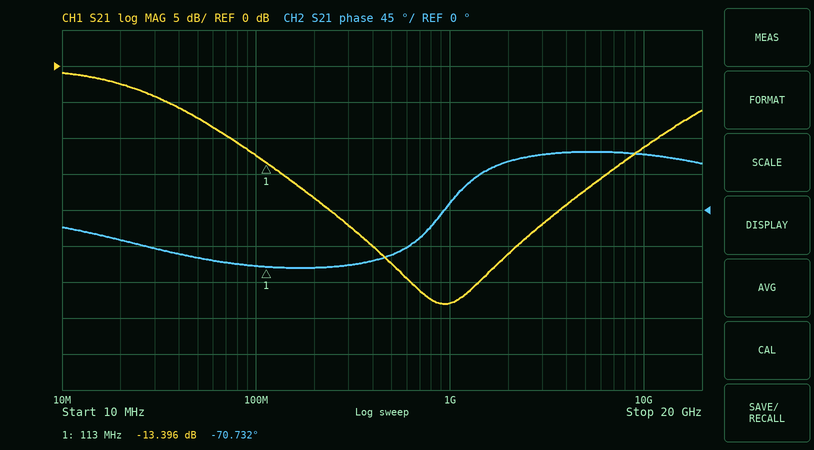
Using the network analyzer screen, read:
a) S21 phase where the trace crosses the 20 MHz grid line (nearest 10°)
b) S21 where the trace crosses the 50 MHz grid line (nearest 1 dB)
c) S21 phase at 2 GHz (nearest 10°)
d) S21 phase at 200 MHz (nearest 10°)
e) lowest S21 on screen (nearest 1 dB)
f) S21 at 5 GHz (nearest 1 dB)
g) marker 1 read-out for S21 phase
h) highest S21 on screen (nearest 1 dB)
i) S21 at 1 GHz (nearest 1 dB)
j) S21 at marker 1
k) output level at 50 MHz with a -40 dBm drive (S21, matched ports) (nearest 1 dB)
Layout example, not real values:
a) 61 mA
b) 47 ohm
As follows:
a) -40°
b) -7 dB
c) 60°
d) -70°
e) -33 dB
f) -17 dB
g) -70.732°
h) -1 dB
i) -33 dB
j) -13.396 dB
k) -47 dBm
